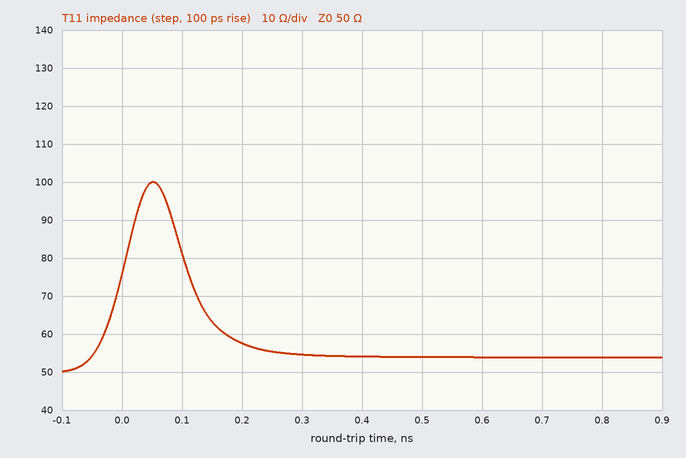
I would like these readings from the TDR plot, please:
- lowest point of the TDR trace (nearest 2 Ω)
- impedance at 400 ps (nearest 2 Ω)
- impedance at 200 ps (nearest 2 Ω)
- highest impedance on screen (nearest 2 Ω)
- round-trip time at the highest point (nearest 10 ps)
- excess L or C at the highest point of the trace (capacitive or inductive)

50 Ω
54 Ω
58 Ω
100 Ω
50 ps
inductive
